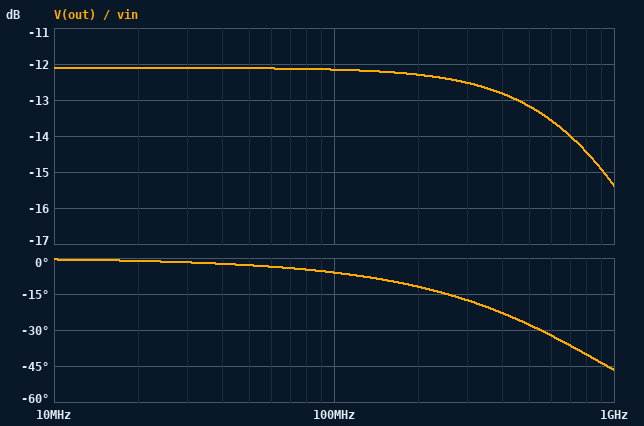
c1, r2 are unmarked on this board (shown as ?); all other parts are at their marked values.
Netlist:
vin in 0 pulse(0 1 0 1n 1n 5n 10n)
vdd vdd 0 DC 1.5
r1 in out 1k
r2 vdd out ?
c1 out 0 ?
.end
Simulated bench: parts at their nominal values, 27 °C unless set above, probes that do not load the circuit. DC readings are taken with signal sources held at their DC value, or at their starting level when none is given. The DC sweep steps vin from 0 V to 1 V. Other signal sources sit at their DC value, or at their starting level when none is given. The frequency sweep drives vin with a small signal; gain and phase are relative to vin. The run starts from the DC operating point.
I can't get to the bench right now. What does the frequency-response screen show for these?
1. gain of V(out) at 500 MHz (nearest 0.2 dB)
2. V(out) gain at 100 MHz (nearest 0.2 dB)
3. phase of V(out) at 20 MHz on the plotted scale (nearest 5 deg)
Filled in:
-13.2 dB
-12.2 dB
0 deg
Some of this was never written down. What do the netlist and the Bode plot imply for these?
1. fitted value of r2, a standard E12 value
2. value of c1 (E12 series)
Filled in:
330 Ω
680 fF
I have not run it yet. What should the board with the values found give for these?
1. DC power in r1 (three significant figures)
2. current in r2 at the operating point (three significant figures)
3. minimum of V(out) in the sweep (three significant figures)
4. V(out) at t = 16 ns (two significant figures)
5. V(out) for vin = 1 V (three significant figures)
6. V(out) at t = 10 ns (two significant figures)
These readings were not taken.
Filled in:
1.27 mW
1.13 mA
1.13 V
1.4 V
1.38 V
1.1 V
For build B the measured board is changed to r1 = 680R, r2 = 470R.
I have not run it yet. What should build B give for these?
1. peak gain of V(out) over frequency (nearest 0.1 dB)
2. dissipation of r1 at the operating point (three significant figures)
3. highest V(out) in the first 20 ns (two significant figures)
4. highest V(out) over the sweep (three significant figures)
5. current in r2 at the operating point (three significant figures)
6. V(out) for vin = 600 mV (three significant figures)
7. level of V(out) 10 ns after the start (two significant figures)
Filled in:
-7.8 dB
1.16 mW
1.3 V
1.30 V
1.30 mA
1.13 V
890 mV
